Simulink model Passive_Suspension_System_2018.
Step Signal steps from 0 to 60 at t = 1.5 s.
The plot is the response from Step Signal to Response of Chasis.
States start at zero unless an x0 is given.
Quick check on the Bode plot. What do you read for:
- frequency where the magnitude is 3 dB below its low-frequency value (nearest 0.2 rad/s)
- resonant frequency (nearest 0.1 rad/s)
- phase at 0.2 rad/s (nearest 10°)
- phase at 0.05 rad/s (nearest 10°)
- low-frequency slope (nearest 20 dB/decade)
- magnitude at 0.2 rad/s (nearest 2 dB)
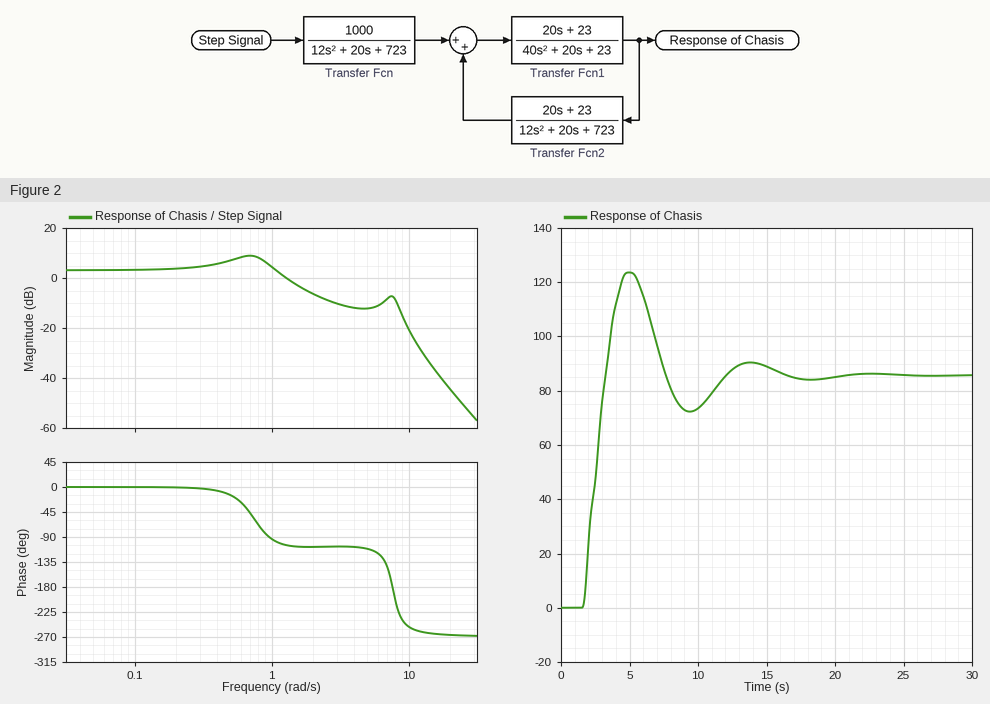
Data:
1.2 rad/s
0.7 rad/s
0°
0°
0 dB/decade
4 dB
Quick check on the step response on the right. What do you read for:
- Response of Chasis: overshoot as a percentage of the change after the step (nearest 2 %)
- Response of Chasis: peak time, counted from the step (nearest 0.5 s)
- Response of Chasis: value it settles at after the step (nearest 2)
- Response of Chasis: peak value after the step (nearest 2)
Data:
44 %
3.5 s
86
124
